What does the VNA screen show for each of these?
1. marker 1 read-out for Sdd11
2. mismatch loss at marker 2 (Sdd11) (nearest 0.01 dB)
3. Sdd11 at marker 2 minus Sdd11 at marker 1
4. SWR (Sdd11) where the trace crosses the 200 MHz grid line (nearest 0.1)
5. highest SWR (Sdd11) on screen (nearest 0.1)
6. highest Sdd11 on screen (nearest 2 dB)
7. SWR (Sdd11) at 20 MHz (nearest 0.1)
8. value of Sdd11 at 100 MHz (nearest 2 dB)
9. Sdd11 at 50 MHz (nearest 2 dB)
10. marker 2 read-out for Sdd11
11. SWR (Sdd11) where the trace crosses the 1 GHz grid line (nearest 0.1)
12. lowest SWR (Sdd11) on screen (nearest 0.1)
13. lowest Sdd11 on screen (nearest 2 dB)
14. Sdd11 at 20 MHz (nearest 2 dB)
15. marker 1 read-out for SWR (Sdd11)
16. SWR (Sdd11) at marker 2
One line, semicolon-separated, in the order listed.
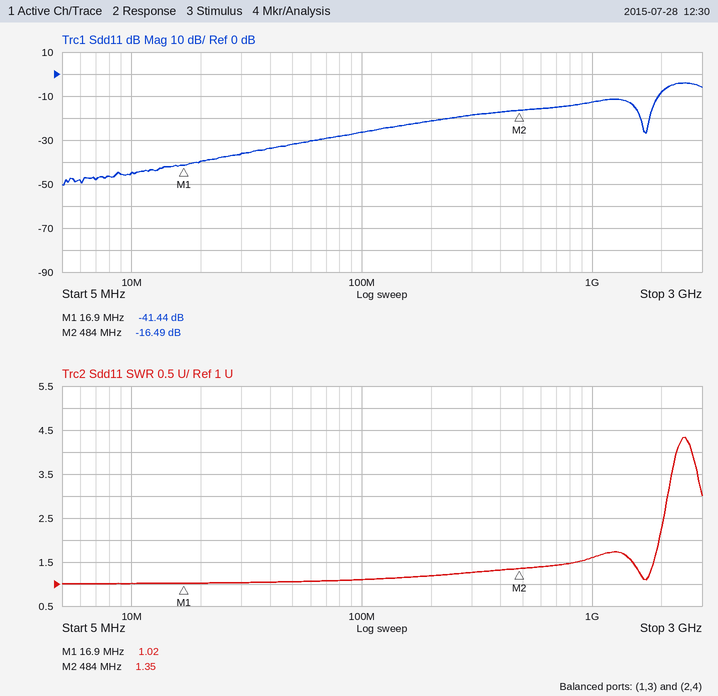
-41.44 dB; 0.10 dB; 24.95 dB; 1.2; 4.3; -4 dB; 1.0; -26 dB; -32 dB; -16.49 dB; 1.6; 1.0; -50 dB; -40 dB; 1.02; 1.35
